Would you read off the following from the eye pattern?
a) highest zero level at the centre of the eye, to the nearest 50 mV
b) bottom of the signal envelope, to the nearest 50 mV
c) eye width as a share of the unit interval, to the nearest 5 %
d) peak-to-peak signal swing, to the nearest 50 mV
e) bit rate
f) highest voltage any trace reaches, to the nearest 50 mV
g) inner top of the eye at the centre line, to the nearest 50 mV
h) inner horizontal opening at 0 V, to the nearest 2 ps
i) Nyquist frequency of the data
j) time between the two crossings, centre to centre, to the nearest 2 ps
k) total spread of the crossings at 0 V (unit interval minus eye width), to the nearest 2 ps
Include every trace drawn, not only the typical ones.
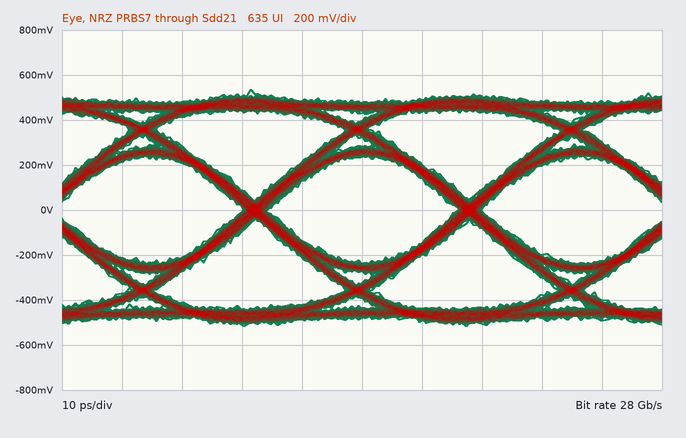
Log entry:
-250 mV
-500 mV
90 %
1.05 V
28 Gb/s
550 mV
250 mV
32 ps
14 GHz
36 ps
4 ps
